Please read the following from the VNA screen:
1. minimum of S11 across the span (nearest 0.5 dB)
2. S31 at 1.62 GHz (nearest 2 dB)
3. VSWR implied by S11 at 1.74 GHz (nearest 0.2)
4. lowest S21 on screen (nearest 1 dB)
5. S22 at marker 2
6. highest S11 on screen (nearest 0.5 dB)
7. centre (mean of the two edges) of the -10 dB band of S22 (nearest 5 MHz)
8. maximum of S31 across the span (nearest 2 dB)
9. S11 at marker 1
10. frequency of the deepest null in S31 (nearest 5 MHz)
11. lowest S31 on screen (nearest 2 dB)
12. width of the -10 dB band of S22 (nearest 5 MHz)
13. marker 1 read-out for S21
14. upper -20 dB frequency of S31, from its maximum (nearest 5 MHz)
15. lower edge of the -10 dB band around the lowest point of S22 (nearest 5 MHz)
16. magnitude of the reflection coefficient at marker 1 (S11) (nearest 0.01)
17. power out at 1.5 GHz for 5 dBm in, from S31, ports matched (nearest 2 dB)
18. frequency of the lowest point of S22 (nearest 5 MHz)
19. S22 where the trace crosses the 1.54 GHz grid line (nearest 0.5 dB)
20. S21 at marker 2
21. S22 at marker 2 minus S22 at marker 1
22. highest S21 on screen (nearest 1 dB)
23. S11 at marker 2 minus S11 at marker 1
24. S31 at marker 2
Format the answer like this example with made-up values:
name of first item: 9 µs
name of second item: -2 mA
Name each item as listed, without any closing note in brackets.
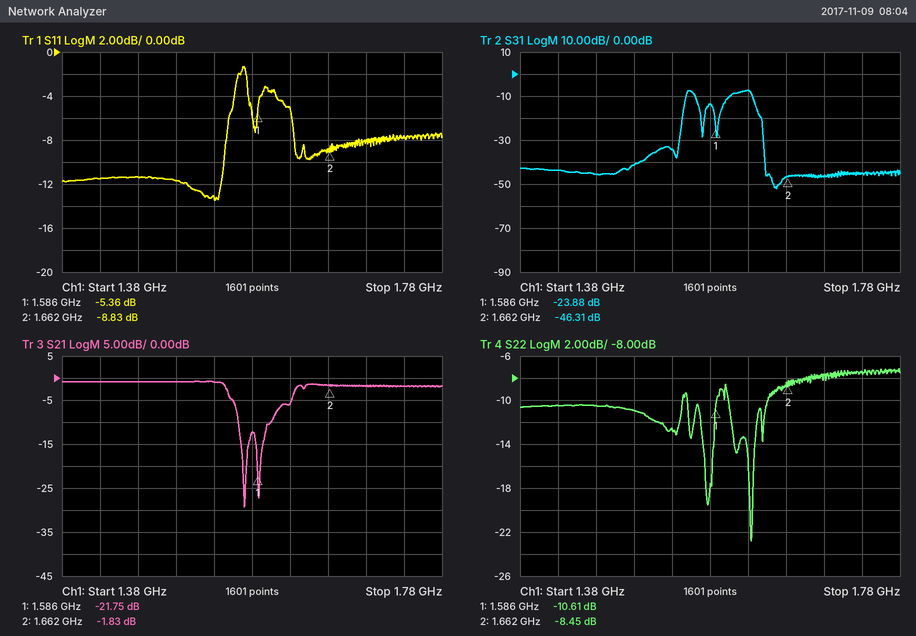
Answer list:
minimum of S11 across the span: -13.5 dB
S31 at 1.62 GHz: -8 dB
VSWR implied by S11 at 1.74 GHz: 2.4
lowest S21 on screen: -29 dB
S22 at marker 2: -8.45 dB
highest S11 on screen: -1.5 dB
centre (mean of the two edges) of the -10 dB band of S22: 1.620 GHz
maximum of S31 across the span: -8 dB
S11 at marker 1: -5.36 dB
frequency of the deepest null in S31: 1.650 GHz
lowest S31 on screen: -52 dB
width of the -10 dB band of S22: 40 MHz
marker 1 read-out for S21: -21.75 dB
upper -20 dB frequency of S31, from its maximum: 1.635 GHz
lower edge of the -10 dB band around the lowest point of S22: 1.600 GHz
magnitude of the reflection coefficient at marker 1 (S11): 0.54
power out at 1.5 GHz for 5 dBm in, from S31, ports matched: -36 dBm
frequency of the lowest point of S22: 1.625 GHz
S22 where the trace crosses the 1.54 GHz grid line: -12.5 dB
S21 at marker 2: -1.83 dB
S22 at marker 2 minus S22 at marker 1: 2.16 dB
highest S21 on screen: -1 dB
S11 at marker 2 minus S11 at marker 1: -3.47 dB
S31 at marker 2: -46.31 dB
